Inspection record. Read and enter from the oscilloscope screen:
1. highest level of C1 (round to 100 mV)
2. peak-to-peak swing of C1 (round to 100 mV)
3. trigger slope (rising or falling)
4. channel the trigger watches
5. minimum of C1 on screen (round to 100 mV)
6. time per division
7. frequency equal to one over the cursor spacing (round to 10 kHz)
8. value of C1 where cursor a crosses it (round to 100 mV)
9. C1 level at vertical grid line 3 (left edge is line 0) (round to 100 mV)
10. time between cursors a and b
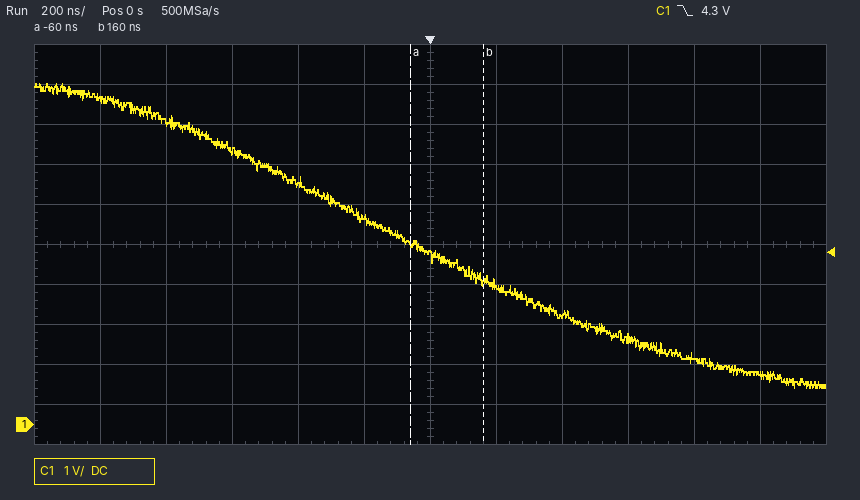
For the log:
8.5 V
7.6 V
falling
C1
900 mV
200 ns
4.55 MHz
4.5 V
6.8 V
220 ns
